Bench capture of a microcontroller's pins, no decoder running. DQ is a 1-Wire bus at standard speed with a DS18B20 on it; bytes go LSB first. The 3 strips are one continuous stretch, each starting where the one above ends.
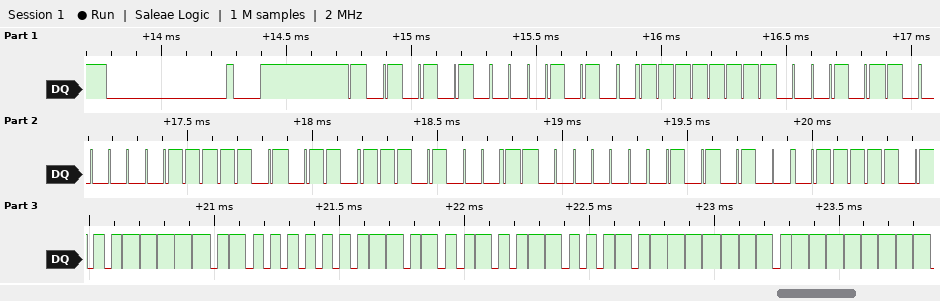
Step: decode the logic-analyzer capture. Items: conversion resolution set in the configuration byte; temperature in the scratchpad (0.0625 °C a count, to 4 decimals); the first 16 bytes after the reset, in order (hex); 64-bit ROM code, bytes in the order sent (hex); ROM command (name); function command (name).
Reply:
12 bits
23.7500 °C
55 28 FF 68 E0 6B 17 03 2A BE 7C 01 4B 46 7F FF
28 FF 68 E0 6B 17 03 2A
Match ROM
Read Scratchpad
